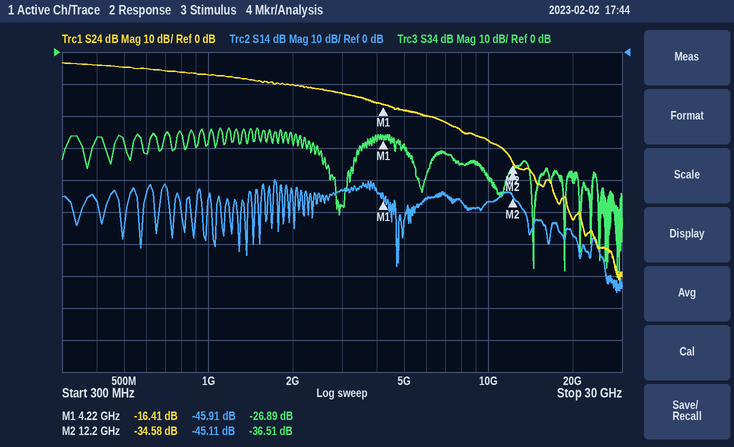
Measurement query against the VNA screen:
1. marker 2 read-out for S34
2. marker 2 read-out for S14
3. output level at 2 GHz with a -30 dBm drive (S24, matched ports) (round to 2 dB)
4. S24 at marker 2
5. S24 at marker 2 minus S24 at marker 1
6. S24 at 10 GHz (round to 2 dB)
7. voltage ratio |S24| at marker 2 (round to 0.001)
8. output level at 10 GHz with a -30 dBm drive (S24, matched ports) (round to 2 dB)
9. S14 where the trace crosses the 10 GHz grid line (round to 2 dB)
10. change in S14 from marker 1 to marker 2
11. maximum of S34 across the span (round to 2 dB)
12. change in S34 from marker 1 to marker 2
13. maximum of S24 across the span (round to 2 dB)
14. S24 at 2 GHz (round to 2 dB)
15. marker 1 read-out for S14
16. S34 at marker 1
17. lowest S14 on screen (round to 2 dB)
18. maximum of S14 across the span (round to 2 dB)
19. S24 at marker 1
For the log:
-36.51 dB
-45.11 dB
-40 dBm
-34.58 dB
-18.17 dB
-28 dB
0.019
-58 dBm
-46 dB
0.80 dB
-24 dB
-9.62 dB
-4 dB
-10 dB
-45.91 dB
-26.89 dB
-76 dB
-40 dB
-16.41 dB
